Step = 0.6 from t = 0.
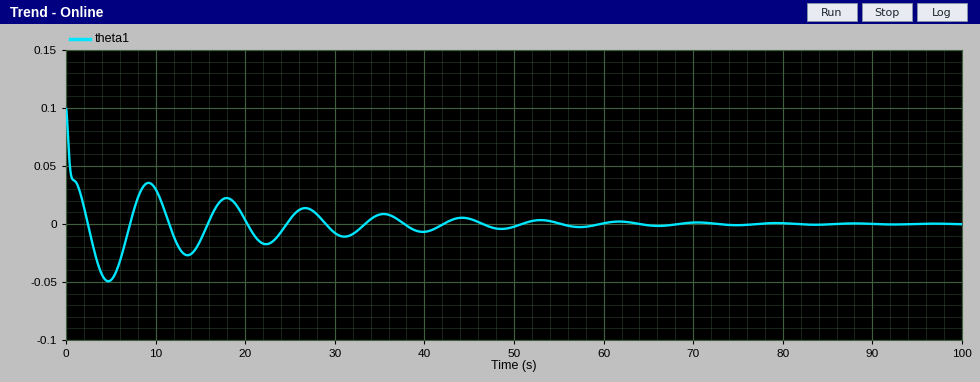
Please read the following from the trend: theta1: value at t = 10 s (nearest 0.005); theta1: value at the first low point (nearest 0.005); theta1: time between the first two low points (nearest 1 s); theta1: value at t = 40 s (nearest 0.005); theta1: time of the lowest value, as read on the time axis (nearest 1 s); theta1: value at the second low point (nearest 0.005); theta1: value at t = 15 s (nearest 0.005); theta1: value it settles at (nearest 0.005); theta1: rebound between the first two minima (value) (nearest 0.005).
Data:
0.030
-0.050
9 s
-0.005
5 s
-0.025
-0.015
0.000
0.035
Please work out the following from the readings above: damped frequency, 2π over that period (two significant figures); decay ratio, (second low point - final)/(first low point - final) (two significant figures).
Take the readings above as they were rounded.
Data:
0.70 rad/s
0.50
